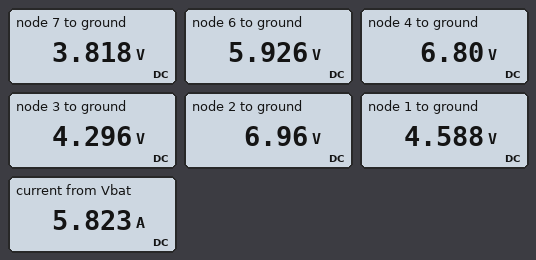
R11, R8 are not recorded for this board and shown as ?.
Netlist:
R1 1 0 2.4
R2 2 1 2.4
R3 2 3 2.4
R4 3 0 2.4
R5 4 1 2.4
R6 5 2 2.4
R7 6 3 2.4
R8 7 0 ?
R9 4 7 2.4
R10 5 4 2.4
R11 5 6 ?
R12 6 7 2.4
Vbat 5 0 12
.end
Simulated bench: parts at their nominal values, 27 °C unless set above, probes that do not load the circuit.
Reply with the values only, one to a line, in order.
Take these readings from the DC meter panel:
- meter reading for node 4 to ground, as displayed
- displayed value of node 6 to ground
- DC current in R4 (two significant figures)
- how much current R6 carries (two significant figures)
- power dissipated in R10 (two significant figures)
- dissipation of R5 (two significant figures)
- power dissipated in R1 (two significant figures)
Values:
6.80 V
5.926 V
1.8 A
2.1 A
11 W
2.0 W
8.8 W
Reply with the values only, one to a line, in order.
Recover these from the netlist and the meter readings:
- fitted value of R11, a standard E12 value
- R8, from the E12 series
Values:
3.9 Ω
1.8 Ω
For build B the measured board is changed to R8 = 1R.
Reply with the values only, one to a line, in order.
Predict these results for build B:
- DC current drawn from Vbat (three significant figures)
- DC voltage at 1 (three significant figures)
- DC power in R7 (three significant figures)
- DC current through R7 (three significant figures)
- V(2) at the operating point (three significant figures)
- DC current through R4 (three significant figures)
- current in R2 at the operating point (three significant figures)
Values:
6.20 A
4.39 V
735 mW
553 mA
6.82 V
1.70 A
1.01 A
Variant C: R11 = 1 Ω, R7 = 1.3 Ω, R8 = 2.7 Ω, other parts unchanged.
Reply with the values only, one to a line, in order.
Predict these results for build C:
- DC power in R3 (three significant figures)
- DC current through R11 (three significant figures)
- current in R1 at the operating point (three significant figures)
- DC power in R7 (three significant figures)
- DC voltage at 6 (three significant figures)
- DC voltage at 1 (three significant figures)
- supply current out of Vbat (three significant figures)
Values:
1.01 W
3.24 A
2.14 A
4.93 W
8.76 V
5.13 V
6.83 A
